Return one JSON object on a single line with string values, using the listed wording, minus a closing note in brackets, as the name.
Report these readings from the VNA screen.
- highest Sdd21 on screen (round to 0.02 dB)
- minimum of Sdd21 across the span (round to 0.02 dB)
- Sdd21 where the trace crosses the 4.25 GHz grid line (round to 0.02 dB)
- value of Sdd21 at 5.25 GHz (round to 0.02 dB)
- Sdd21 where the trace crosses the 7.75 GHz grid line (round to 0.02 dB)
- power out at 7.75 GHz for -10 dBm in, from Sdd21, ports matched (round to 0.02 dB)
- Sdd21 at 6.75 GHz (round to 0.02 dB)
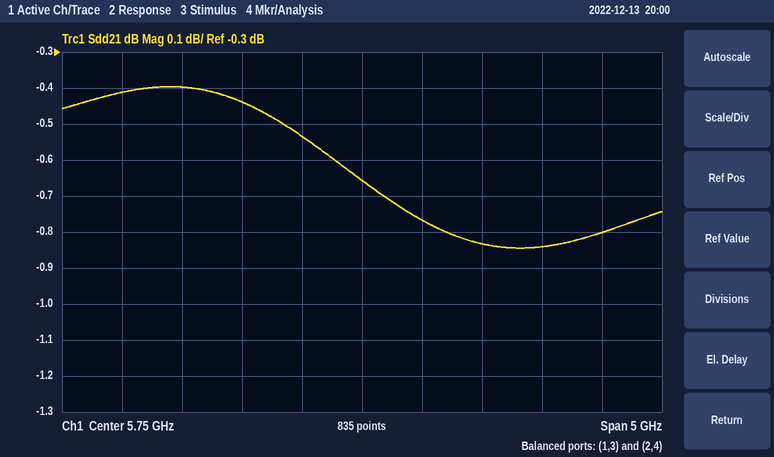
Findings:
{"highest Sdd21 on screen": "-0.40 dB", "minimum of Sdd21 across the span": "-0.84 dB", "Sdd21 where the trace crosses the 4.25 GHz grid line": "-0.40 dB", "value of Sdd21 at 5.25 GHz": "-0.54 dB", "Sdd21 where the trace crosses the 7.75 GHz grid line": "-0.80 dB", "power out at 7.75 GHz for -10 dBm in, from Sdd21, ports matched": "-10.80 dBm", "Sdd21 at 6.75 GHz": "-0.84 dB"}
